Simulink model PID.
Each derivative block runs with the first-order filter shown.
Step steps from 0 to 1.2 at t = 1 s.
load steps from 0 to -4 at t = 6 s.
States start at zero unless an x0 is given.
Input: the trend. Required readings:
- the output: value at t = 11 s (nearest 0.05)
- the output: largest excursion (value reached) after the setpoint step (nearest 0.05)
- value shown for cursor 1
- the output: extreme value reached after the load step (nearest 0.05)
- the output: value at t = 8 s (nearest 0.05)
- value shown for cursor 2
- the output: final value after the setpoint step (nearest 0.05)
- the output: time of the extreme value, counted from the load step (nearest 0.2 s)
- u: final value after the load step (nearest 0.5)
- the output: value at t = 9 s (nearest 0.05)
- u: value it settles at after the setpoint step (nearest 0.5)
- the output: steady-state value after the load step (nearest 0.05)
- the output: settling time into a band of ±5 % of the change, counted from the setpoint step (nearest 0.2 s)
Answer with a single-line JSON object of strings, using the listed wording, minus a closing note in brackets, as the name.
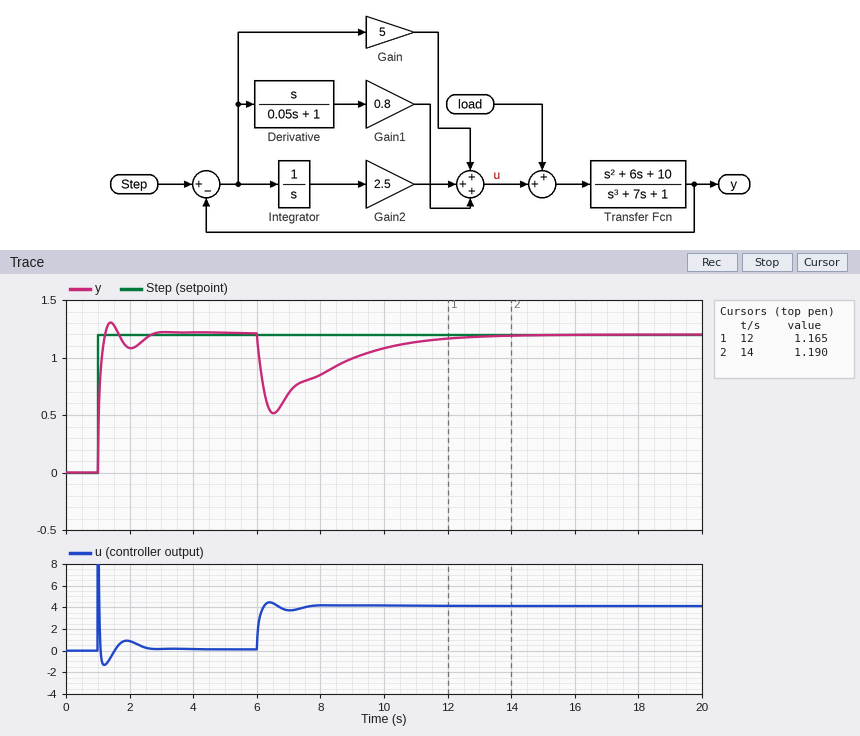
{"the output: value at t = 11 s": "1.15", "the output: largest excursion (value reached) after the setpoint step": "1.30", "value shown for cursor 1": "1.165", "the output: extreme value reached after the load step": "0.50", "the output: value at t = 8 s": "0.85", "value shown for cursor 2": "1.190", "the output: final value after the setpoint step": "1.20", "the output: time of the extreme value, counted from the load step": "0.6 s", "u: final value after the load step": "4.0", "the output: value at t = 9 s": "1.00", "u: value it settles at after the setpoint step": "0.0", "the output: steady-state value after the load step": "1.20", "the output: settling time into a band of ±5 % of the change, counted from the setpoint step": "1.4 s"}
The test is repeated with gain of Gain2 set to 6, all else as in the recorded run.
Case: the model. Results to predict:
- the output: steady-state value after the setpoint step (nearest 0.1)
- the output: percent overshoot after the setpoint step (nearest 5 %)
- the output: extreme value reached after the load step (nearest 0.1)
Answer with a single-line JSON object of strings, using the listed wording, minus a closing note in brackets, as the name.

{"the output: steady-state value after the setpoint step": "1.2", "the output: percent overshoot after the setpoint step": "10 %", "the output: extreme value reached after the load step": "0.6"}
